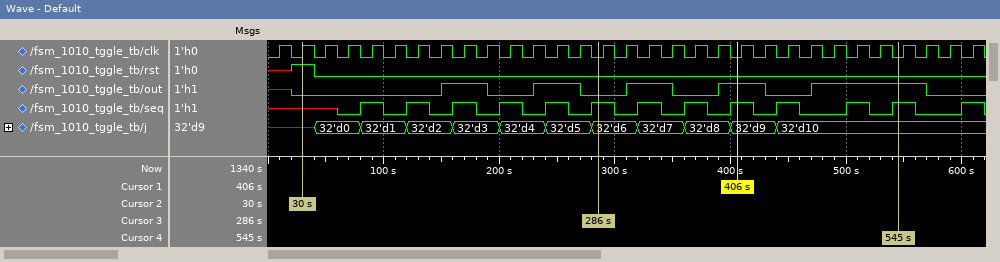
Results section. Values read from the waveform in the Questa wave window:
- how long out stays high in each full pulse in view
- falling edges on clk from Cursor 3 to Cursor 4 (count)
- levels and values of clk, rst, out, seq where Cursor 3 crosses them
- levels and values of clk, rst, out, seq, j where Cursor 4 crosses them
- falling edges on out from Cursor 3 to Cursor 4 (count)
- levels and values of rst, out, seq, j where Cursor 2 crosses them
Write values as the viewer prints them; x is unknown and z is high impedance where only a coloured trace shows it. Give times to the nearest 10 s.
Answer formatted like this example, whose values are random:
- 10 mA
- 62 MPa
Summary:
- 40 s, 40 s, 40 s, 40 s, 100 s
- 13
- clk=0, rst=0, out=0, seq=1
- clk=0, rst=0, out=1, seq=1, j=32'd10
- 2
- rst=1, out=0, seq=x, j=x
